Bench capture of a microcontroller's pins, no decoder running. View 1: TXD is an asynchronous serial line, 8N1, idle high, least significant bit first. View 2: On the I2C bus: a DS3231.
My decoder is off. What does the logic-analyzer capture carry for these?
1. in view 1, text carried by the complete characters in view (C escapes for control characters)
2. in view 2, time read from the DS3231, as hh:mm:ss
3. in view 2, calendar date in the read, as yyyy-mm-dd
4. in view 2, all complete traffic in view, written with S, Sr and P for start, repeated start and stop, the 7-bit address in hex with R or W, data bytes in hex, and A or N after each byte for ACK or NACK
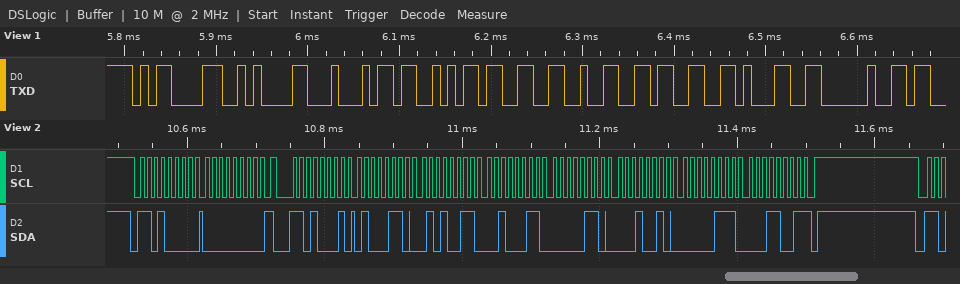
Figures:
"\r\nDS3231 "
23:53:46
2019-07-12
S 68W A 00 A Sr 68R A 46 A 53 A 23 A 06 A 12 A 07 A 19 N P
